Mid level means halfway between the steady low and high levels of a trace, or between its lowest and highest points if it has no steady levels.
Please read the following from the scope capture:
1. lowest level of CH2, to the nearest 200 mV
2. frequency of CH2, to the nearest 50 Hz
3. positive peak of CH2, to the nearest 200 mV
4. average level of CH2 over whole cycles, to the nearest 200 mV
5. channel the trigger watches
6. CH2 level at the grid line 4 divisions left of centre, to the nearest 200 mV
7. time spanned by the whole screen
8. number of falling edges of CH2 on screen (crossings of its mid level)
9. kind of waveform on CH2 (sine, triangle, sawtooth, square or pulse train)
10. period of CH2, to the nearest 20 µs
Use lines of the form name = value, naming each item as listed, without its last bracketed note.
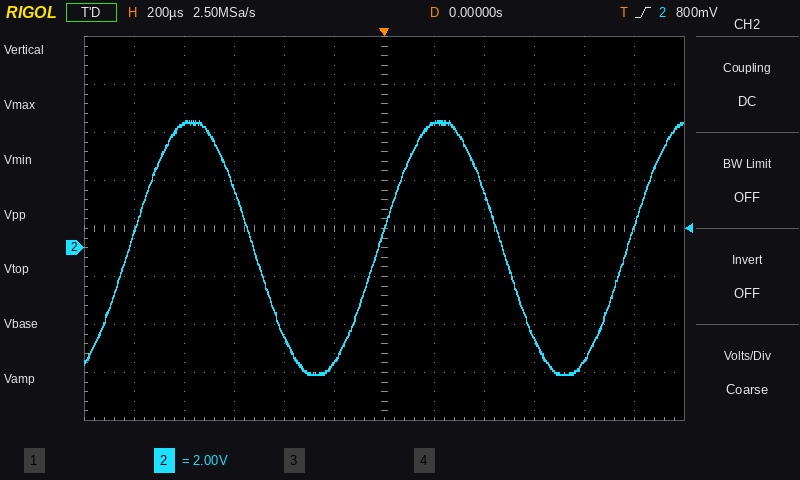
lowest level of CH2, to the nearest 200 mV = -5.2 V
frequency of CH2, to the nearest 50 Hz = 1.00 kHz
positive peak of CH2, to the nearest 200 mV = 5.2 V
average level of CH2 over whole cycles, to the nearest 200 mV = 0.0 V
channel the trigger watches = CH2
CH2 level at the grid line 4 divisions left of centre, to the nearest 200 mV = 5.2 V
time spanned by the whole screen = 2.4 ms
number of falling edges of CH2 on screen = 2
kind of waveform on CH2 = sine
period of CH2, to the nearest 20 µs = 1.00 ms
